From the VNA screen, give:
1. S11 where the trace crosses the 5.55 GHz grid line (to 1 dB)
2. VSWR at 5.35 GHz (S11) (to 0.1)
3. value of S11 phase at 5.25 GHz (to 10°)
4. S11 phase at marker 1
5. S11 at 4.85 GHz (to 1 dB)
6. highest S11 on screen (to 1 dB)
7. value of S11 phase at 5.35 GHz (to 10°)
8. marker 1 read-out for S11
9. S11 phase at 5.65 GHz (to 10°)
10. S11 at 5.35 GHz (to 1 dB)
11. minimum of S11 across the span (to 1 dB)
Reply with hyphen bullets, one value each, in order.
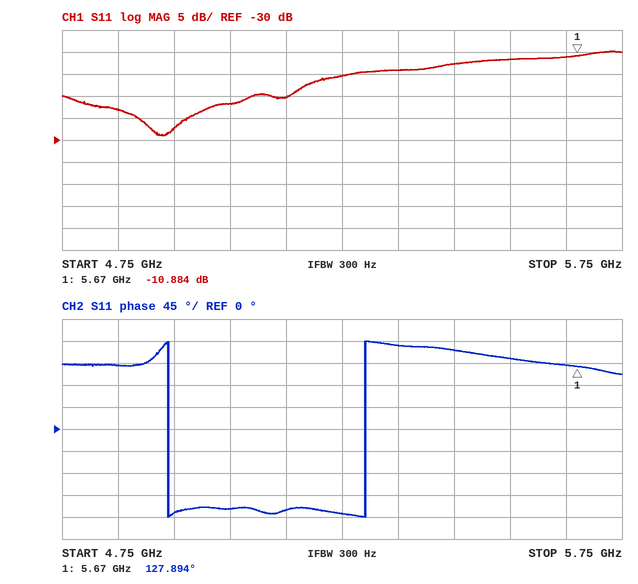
- -12 dB
- 1.5
- -170°
- 127.894°
- -23 dB
- -10 dB
- 170°
- -10.884 dB
- 130°
- -14 dB
- -29 dB
